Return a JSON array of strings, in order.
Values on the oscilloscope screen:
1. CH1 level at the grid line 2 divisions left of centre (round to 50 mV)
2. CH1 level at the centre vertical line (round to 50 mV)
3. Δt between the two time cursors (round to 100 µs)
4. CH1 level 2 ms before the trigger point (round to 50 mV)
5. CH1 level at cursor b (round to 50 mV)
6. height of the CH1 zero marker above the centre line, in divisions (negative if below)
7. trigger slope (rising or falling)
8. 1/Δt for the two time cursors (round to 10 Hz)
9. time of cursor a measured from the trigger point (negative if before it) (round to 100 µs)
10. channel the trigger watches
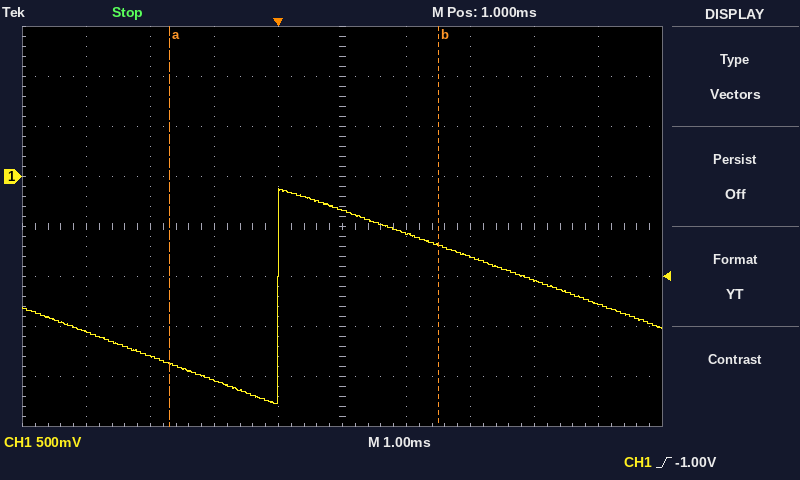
["-2.05 V", "-350 mV", "4.2 ms", "-1.80 V", "-700 mV", "+1.0 div", "rising", "240 Hz", "-1.7 ms", "CH1"]
